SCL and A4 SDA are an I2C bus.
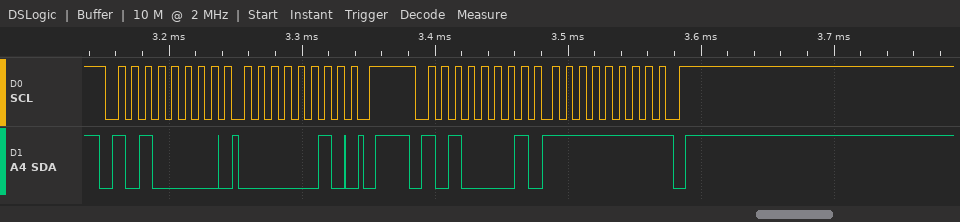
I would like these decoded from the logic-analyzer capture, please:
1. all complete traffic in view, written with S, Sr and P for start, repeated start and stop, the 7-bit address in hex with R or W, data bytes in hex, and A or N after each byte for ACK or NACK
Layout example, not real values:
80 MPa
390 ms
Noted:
S 50W A 02 A P S 50R A FF N P
